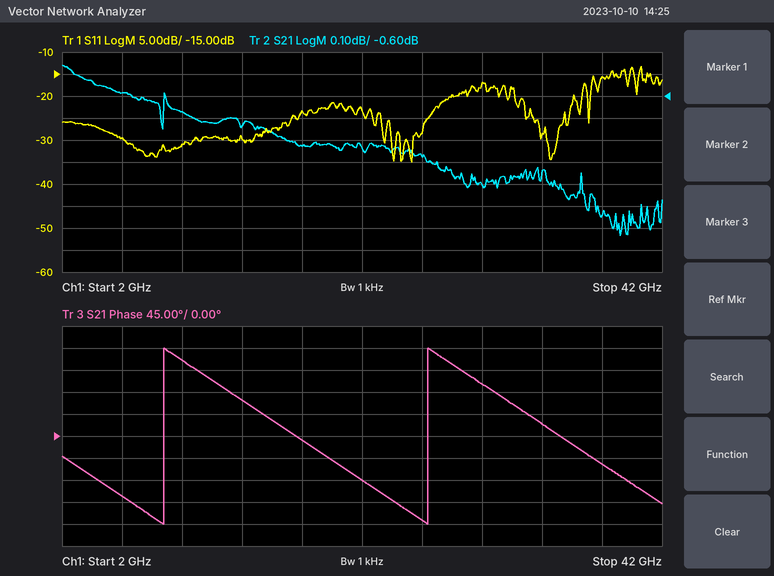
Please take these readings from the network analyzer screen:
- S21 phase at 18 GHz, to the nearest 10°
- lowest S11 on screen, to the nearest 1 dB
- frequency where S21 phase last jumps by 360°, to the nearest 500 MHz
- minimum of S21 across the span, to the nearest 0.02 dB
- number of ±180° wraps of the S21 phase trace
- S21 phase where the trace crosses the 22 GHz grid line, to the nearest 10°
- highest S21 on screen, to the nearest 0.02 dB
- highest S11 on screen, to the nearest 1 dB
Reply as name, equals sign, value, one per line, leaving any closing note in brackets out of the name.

S21 phase at 18 GHz, to the nearest 10° = -10°
lowest S11 on screen, to the nearest 1 dB = -35 dB
frequency where S21 phase last jumps by 360°, to the nearest 500 MHz = 26.5 GHz
minimum of S21 across the span, to the nearest 0.02 dB = -1.24 dB
number of ±180° wraps of the S21 phase trace = 2
S21 phase where the trace crosses the 22 GHz grid line, to the nearest 10° = -90°
highest S21 on screen, to the nearest 0.02 dB = -0.46 dB
highest S11 on screen, to the nearest 1 dB = -13 dB
